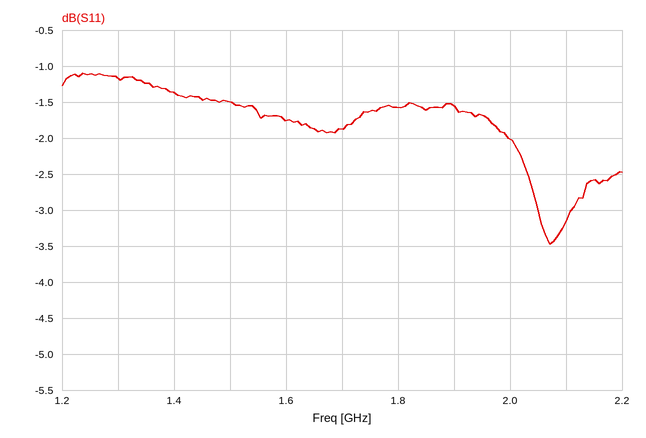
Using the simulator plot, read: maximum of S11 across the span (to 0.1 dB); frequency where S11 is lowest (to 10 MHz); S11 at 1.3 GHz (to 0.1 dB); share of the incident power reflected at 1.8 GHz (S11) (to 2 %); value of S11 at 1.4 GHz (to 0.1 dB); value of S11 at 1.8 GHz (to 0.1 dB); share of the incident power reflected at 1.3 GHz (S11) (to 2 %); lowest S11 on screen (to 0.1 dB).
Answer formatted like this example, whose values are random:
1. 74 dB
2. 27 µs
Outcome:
1. -1.1 dB
2. 2.07 GHz
3. -1.2 dB
4. 70 %
5. -1.4 dB
6. -1.6 dB
7. 76 %
8. -3.5 dB
